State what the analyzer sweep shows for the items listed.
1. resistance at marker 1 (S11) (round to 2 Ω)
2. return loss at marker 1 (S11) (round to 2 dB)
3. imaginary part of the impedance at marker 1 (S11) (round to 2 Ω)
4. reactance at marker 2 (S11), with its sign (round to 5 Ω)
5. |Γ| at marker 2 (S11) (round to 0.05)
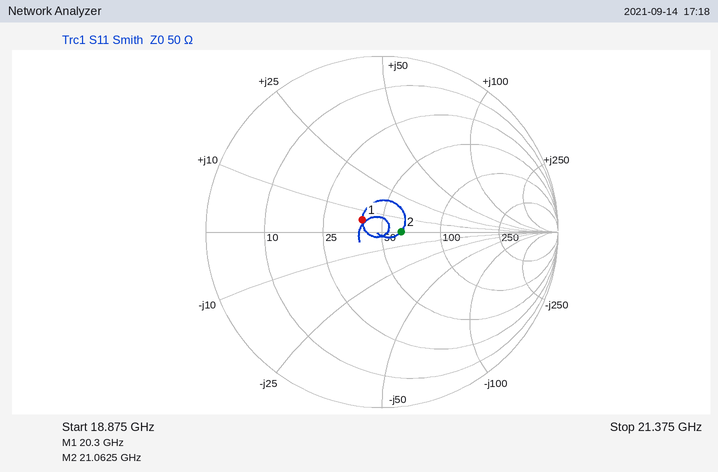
40 Ω
18 dB
+6 Ω
0 Ω
0.10
